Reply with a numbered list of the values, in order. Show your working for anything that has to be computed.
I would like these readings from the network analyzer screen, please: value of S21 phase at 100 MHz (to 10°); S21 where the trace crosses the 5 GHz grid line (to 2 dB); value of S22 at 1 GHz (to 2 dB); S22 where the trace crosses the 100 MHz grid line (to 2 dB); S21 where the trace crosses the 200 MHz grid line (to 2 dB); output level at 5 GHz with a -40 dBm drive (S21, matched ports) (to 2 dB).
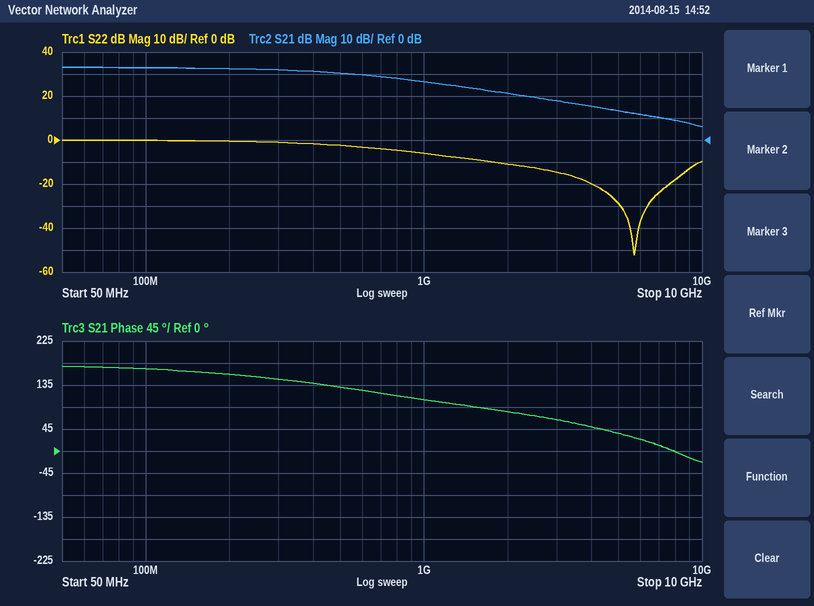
1. 170°
2. 14 dB
3. -6 dB
4. 0 dB
5. 32 dB
6. -40 dBm + (14 dB) = -26 dBm
